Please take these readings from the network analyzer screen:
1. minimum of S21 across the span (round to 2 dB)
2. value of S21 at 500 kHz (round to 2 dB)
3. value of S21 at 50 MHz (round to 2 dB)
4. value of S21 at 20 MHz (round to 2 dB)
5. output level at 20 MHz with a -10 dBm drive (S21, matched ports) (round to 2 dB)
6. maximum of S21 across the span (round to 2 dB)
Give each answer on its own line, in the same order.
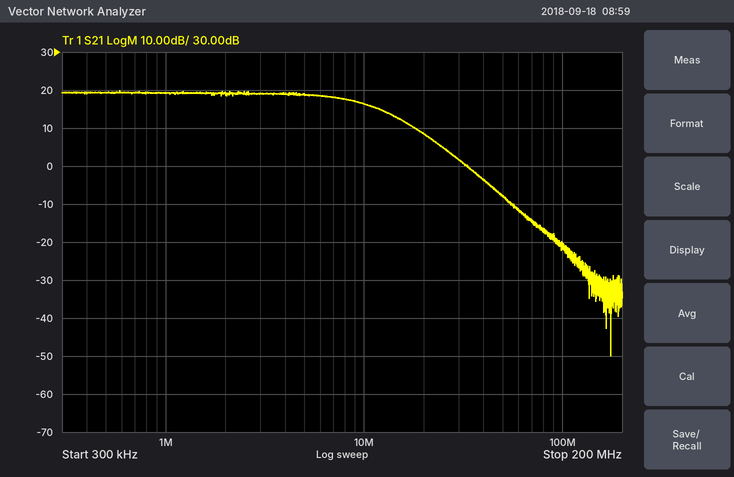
-50 dB
20 dB
-8 dB
8 dB
-2 dBm
20 dB
